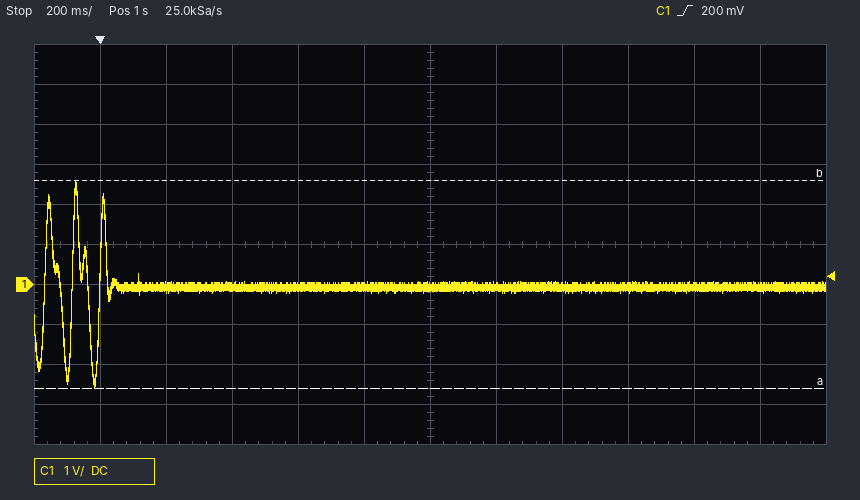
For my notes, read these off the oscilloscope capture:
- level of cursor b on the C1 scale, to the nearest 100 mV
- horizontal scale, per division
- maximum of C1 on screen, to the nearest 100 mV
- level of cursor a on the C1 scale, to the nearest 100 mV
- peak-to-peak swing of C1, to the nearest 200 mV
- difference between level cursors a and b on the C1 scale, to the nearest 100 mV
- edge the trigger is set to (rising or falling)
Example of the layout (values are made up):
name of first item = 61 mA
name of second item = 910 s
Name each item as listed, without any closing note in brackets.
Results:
level of cursor b on the C1 scale, to the nearest 100 mV = 2.6 V
horizontal scale, per division = 200 ms
maximum of C1 on screen, to the nearest 100 mV = 2.6 V
level of cursor a on the C1 scale, to the nearest 100 mV = -2.6 V
peak-to-peak swing of C1, to the nearest 200 mV = 5.2 V
difference between level cursors a and b on the C1 scale, to the nearest 100 mV = 5.2 V
edge the trigger is set to = rising
